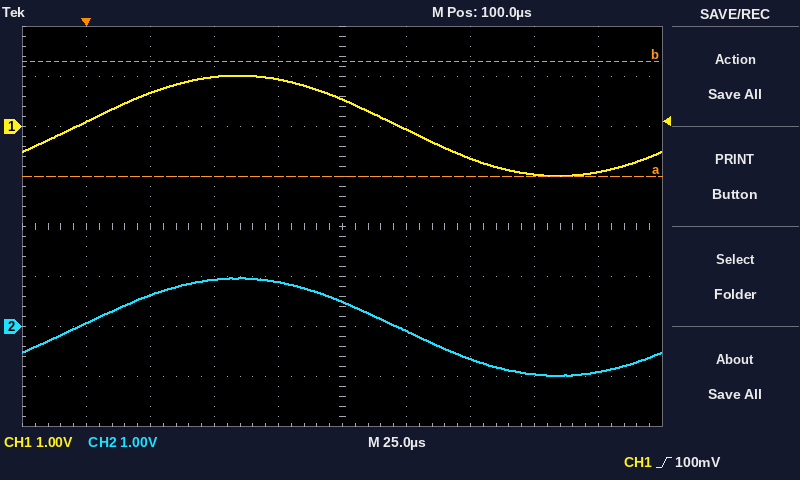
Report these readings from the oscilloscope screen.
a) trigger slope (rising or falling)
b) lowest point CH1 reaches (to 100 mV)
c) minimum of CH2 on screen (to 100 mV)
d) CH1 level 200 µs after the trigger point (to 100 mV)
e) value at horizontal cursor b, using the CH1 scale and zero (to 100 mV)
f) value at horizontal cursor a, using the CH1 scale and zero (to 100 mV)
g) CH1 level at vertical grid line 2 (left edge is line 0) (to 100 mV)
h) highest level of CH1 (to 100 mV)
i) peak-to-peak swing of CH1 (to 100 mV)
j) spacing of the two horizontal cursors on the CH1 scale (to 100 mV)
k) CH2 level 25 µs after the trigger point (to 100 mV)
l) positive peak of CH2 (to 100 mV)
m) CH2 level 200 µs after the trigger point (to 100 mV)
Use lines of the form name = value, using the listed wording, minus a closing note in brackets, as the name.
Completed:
trigger slope = rising
lowest point CH1 reaches = -1.0 V
minimum of CH2 on screen = -1.0 V
CH1 level 200 µs after the trigger point = -900 mV
value at horizontal cursor b, using the CH1 scale and zero = 1.3 V
value at horizontal cursor a, using the CH1 scale and zero = -1.0 V
CH1 level at vertical grid line 2 (left edge is line 0) = 700 mV
highest level of CH1 = 1.0 V
peak-to-peak swing of CH1 = 2.0 V
spacing of the two horizontal cursors on the CH1 scale = 2.3 V
CH2 level 25 µs after the trigger point = 600 mV
positive peak of CH2 = 1.0 V
CH2 level 200 µs after the trigger point = -900 mV
